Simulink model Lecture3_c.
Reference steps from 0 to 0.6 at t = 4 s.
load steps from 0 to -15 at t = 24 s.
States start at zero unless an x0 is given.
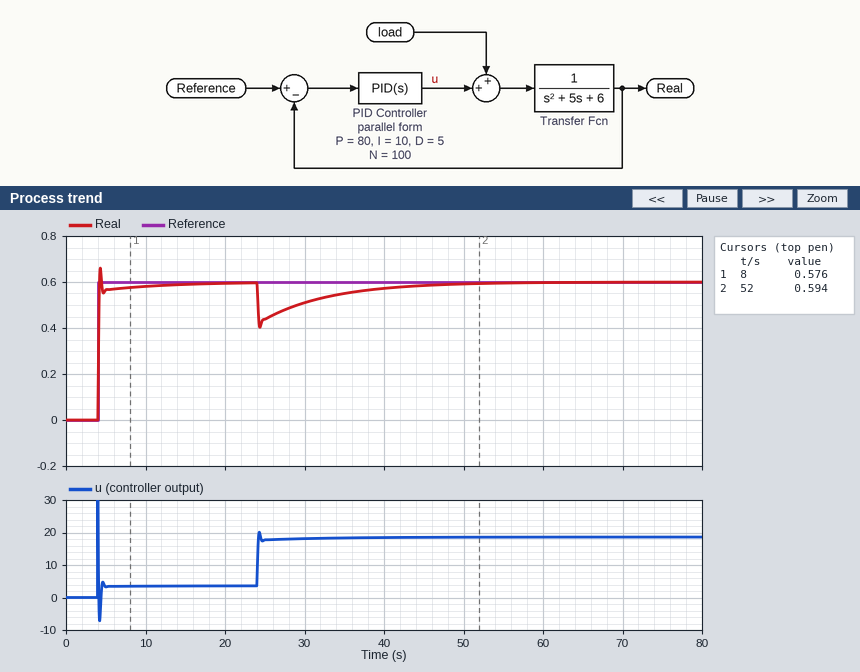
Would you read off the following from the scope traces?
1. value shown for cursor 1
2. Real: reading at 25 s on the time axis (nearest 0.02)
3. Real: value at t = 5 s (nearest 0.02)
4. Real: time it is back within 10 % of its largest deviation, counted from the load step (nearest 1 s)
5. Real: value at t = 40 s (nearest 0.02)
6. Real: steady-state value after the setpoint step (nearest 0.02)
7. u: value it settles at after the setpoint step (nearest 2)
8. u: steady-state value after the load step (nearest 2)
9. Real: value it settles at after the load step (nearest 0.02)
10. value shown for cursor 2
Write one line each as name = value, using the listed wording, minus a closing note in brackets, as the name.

value shown for cursor 1 = 0.576
Real: reading at 25 s on the time axis = 0.44
Real: value at t = 5 s = 0.56
Real: time it is back within 10 % of its largest deviation, counted from the load step = 19 s
Real: value at t = 40 s = 0.58
Real: steady-state value after the setpoint step = 0.60
u: value it settles at after the setpoint step = 4
u: steady-state value after the load step = 18
Real: value it settles at after the load step = 0.60
value shown for cursor 2 = 0.594
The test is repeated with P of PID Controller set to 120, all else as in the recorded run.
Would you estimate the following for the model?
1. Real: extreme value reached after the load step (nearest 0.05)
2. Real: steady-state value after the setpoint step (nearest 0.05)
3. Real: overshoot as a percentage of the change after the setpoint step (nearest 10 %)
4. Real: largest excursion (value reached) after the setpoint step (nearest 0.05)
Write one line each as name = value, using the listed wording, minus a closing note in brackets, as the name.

Real: extreme value reached after the load step = 0.45
Real: steady-state value after the setpoint step = 0.60
Real: overshoot as a percentage of the change after the setpoint step = 20 %
Real: largest excursion (value reached) after the setpoint step = 0.70
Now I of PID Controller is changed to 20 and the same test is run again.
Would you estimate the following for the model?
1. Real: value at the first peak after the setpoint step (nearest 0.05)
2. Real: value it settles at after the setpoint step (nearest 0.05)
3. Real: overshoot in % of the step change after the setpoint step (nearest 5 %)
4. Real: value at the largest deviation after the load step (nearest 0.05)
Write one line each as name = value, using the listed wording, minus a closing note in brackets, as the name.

Real: value at the first peak after the setpoint step = 0.65
Real: value it settles at after the setpoint step = 0.60
Real: overshoot in % of the step change after the setpoint step = 10 %
Real: value at the largest deviation after the load step = 0.40
